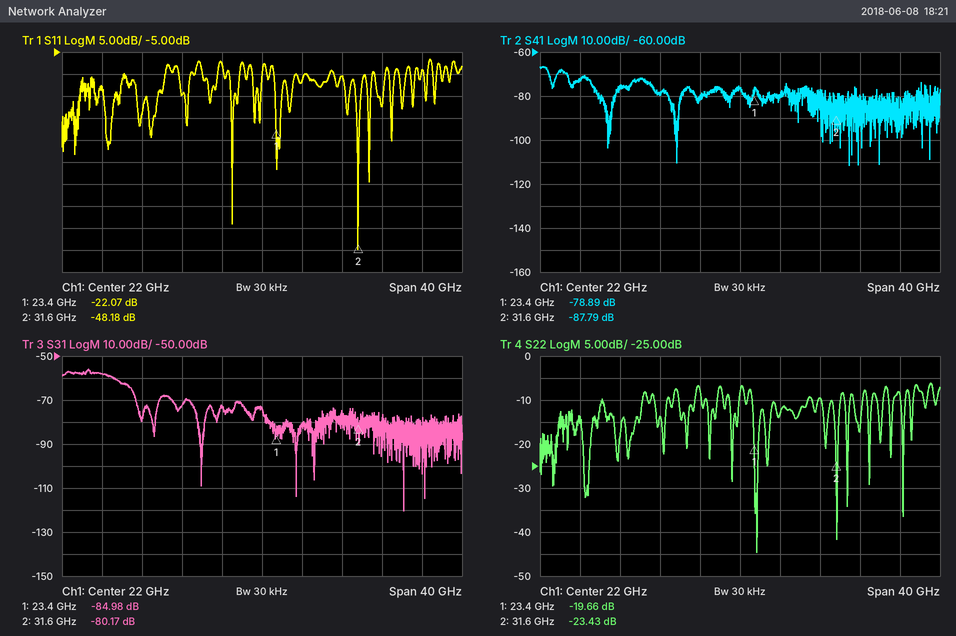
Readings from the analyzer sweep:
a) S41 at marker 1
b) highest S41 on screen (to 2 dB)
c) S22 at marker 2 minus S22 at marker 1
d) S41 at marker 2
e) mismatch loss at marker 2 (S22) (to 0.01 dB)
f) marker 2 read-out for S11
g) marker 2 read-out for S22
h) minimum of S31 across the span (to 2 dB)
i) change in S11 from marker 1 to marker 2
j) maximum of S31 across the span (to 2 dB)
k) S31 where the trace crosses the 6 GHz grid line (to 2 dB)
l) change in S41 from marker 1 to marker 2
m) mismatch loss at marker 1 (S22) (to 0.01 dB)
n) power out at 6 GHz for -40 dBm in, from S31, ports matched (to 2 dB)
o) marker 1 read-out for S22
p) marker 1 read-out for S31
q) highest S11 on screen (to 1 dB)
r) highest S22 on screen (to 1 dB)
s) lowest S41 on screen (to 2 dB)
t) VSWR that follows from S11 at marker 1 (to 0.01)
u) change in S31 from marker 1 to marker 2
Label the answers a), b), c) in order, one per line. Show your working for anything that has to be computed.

a) -78.89 dB
b) -66 dB
c) -23.43 − (-19.66) = -3.77 dB
d) -87.79 dB
e) −10 log10(1 − 10^(-23.43/10)) ≈ 0.02 dB
f) -48.18 dB
g) -23.43 dB
h) -120 dB
i) -48.18 − (-22.07) = -26.11 dB
j) -56 dB
k) -58 dB
l) -87.79 − (-78.89) = -8.90 dB
m) −10 log10(1 − 10^(-19.66/10)) ≈ 0.05 dB
n) -40 dBm + (-58 dB) = -98 dBm
o) -19.66 dB
p) -84.98 dB
q) -7 dB
r) -6 dB
s) -112 dB
t) (1 + 0.0788)/(1 − 0.0788) ≈ 1.17
u) -80.17 − (-84.98) = 4.81 dB
